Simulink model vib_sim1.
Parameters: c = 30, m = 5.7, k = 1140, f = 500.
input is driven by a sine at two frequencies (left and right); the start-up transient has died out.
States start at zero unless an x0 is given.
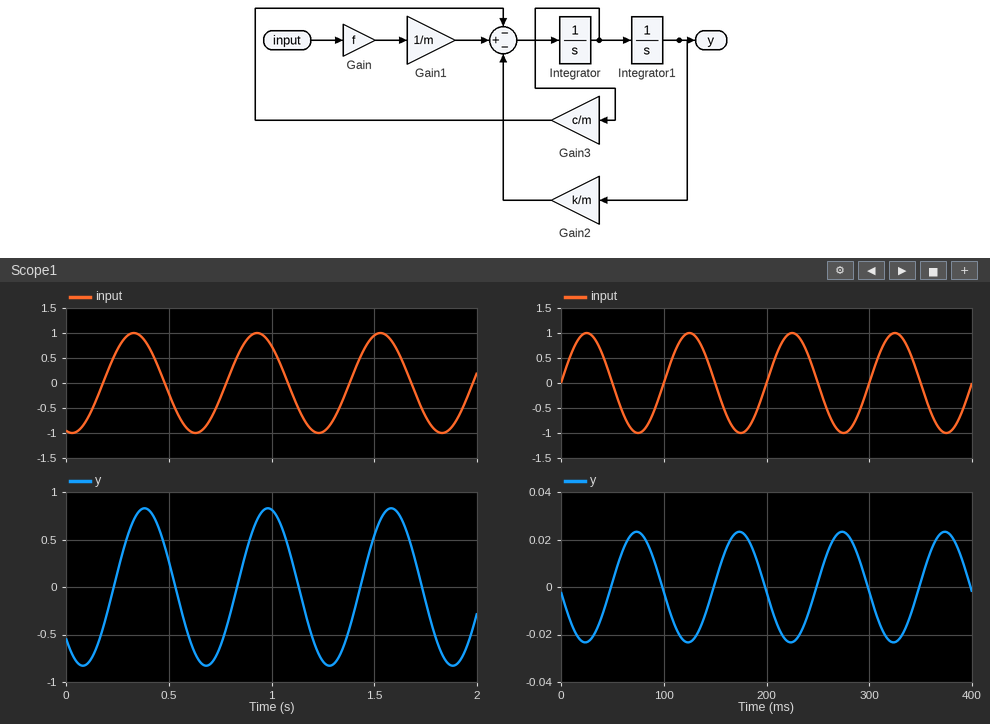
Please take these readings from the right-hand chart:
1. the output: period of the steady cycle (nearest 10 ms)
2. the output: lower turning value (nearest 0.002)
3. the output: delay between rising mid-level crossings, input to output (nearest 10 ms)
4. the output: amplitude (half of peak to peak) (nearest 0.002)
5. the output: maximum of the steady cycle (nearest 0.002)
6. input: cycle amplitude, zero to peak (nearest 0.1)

100 ms
-0.024
50 ms
0.024
0.024
1.0
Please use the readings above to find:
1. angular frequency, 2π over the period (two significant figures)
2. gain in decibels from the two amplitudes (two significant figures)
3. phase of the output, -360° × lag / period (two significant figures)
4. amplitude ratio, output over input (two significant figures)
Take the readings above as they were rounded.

0.063 rad/ms
-32 dB
-180°
0.024
